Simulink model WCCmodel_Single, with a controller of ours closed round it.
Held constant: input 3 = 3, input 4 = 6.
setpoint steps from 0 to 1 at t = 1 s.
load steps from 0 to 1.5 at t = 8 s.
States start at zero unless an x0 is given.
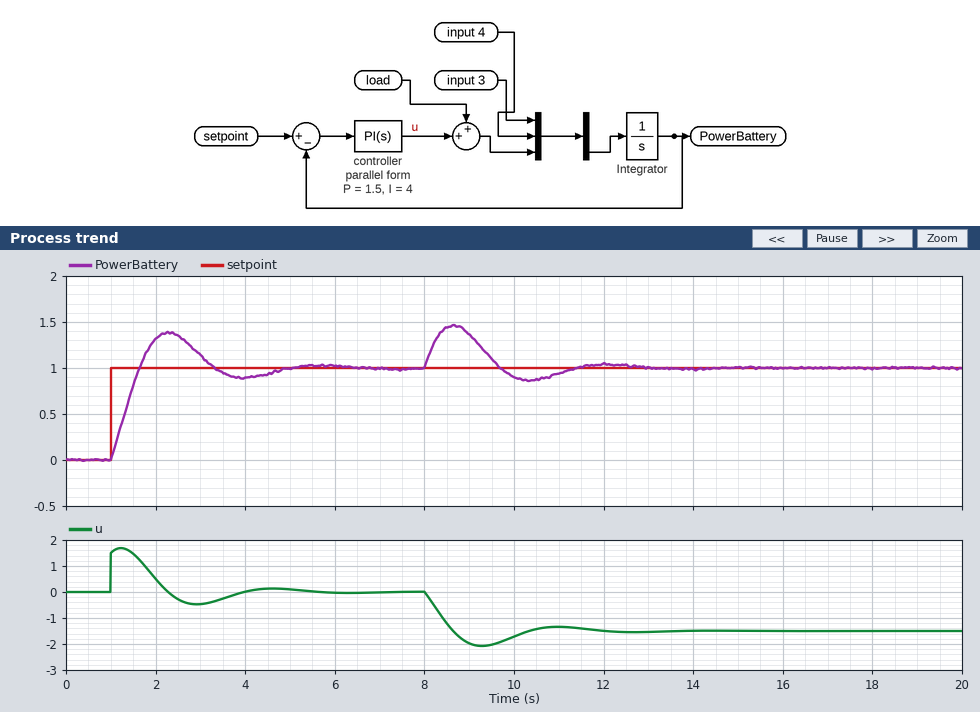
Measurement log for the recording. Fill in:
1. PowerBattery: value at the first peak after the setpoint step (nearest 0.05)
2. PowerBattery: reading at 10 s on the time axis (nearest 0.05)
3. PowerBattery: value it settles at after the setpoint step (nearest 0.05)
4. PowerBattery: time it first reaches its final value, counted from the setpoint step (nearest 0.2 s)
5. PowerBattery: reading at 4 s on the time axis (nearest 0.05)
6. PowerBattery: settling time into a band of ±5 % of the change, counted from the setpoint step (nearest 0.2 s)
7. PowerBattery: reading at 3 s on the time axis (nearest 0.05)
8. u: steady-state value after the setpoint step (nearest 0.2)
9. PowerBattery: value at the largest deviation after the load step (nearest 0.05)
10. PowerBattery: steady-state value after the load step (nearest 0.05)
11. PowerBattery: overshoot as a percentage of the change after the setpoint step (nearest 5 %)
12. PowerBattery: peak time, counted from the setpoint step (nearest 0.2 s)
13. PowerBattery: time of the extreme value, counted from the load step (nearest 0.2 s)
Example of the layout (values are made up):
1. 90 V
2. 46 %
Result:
1. 1.40
2. 0.90
3. 1.00
4. 0.6 s
5. 0.90
6. 3.6 s
7. 1.15
8. 0.0
9. 1.45
10. 1.00
11. 40 %
12. 1.2 s
13. 0.6 s
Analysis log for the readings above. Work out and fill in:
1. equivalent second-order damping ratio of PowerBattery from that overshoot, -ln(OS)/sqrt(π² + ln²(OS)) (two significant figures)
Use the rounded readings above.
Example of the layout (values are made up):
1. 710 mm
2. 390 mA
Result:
1. 0.28
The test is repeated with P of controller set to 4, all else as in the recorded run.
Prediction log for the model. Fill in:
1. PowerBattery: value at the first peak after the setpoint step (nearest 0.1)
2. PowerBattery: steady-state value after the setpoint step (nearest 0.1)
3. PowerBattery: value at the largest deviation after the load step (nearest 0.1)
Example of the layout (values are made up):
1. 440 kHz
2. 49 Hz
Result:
1. 1.1
2. 1.0
3. 1.3
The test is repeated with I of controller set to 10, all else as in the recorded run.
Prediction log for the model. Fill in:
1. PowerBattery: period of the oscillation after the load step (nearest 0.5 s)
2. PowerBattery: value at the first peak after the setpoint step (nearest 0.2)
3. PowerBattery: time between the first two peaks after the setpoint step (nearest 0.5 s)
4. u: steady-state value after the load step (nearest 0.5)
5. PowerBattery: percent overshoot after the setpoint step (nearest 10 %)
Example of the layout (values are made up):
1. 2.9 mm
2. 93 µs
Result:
1. 2.0 s
2. 1.6
3. 2.0 s
4. -1.5
5. 50 %
